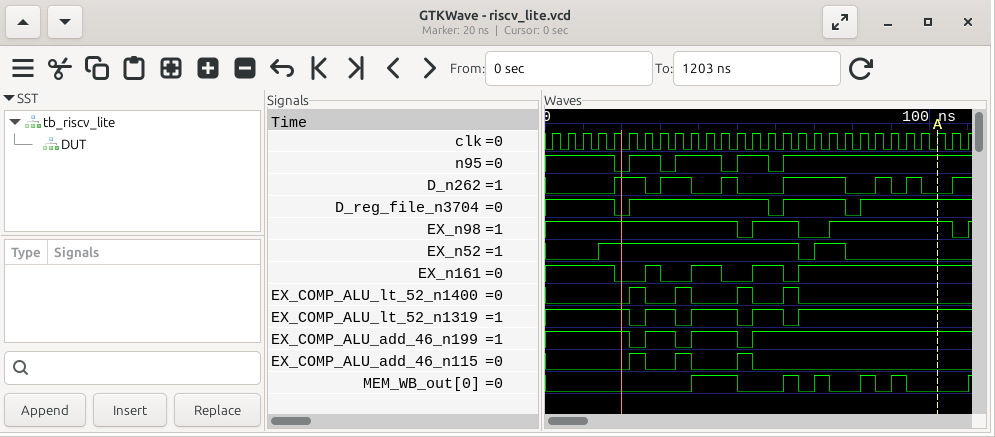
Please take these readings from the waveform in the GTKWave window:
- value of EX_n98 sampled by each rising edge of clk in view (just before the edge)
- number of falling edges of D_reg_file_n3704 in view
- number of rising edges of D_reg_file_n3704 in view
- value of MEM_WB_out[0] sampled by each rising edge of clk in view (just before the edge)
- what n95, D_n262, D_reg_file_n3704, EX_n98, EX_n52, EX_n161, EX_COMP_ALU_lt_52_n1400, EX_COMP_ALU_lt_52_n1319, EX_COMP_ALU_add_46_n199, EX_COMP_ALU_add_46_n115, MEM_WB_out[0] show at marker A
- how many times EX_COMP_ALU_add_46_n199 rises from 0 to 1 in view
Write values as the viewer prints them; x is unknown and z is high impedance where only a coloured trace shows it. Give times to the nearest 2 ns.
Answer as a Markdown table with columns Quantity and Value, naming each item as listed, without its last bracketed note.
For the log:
| Quantity | Value |
|---|---|
| value of EX_n98 sampled by each rising edge of clk in view | 1 1 1 1 1 1 1 1 1 1 1 1 1 0 1 1 1 0 0 1 1 1 1 1 1 1 1 0 |
| number of falling edges of D_reg_file_n3704 in view | 3 |
| number of rising edges of D_reg_file_n3704 in view | 3 |
| value of MEM_WB_out[0] sampled by each rising edge of clk in view | 0 0 0 0 0 0 0 0 0 0 1 1 1 0 0 0 1 0 1 0 0 1 0 1 0 0 0 0 |
| what n95, D_n262, D_reg_file_n3704, EX_n98, EX_n52, EX_n161, EX_COMP_ALU_lt_52_n1400, EX_COMP_ALU_lt_52_n1319, EX_COMP_ALU_add_46_n199, EX_COMP_ALU_add_46_n115, MEM_WB_out[0] show at marker A | n95=1, D_n262=0, D_reg_file_n3704=1, EX_n98=1, EX_n52=0, EX_n161=1, EX_COMP_ALU_lt_52_n1400=0, EX_COMP_ALU_lt_52_n1319=1, EX_COMP_ALU_add_46_n199=1, EX_COMP_ALU_add_46_n115=0, MEM_WB_out[0]=0 |
| how many times EX_COMP_ALU_add_46_n199 rises from 0 to 1 in view | 3 |
